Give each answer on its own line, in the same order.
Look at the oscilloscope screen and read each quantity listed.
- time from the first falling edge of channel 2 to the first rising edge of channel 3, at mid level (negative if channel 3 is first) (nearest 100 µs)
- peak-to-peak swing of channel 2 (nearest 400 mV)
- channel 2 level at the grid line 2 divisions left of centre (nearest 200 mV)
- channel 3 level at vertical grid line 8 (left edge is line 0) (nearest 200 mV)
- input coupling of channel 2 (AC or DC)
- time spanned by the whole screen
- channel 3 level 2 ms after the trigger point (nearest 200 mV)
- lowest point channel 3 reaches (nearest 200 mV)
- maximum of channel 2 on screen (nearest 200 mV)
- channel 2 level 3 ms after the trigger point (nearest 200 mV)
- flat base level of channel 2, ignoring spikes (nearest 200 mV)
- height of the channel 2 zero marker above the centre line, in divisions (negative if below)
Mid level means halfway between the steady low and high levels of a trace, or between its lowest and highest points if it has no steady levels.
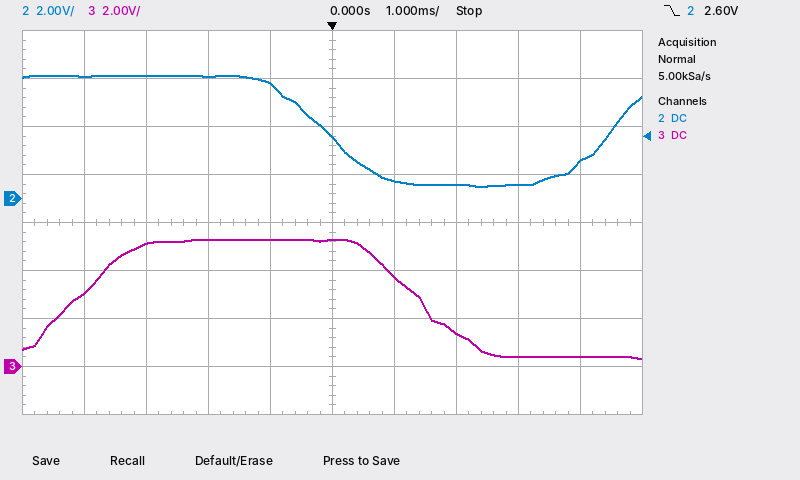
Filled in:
-4.0 ms
4.8 V
5.0 V
400 mV
DC
10 ms
1.4 V
400 mV
5.2 V
600 mV
600 mV
+0.5 div
